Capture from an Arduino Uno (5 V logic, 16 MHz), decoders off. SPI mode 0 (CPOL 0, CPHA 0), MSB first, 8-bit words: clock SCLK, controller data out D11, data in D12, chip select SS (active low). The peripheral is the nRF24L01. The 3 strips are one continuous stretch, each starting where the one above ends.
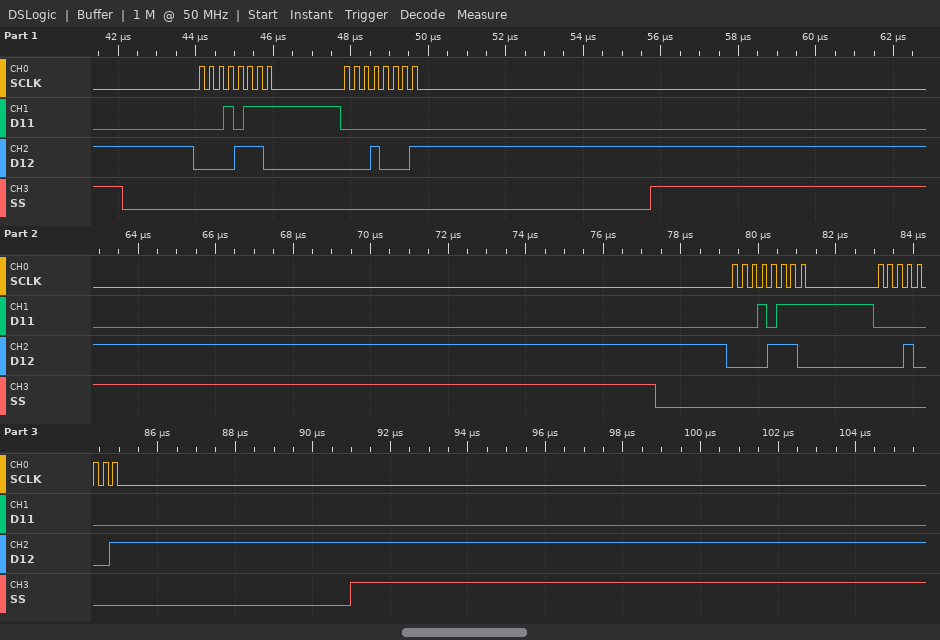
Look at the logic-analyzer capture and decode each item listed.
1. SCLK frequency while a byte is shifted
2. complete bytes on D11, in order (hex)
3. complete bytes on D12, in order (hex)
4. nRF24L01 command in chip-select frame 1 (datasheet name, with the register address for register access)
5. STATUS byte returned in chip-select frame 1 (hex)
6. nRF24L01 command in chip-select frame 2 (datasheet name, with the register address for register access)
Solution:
4 MHz
0x17 0x00 0x17 0x00
0x0E 0x11 0x0E 0x11
R_REGISTER 0x17
0x0E
R_REGISTER 0x17
